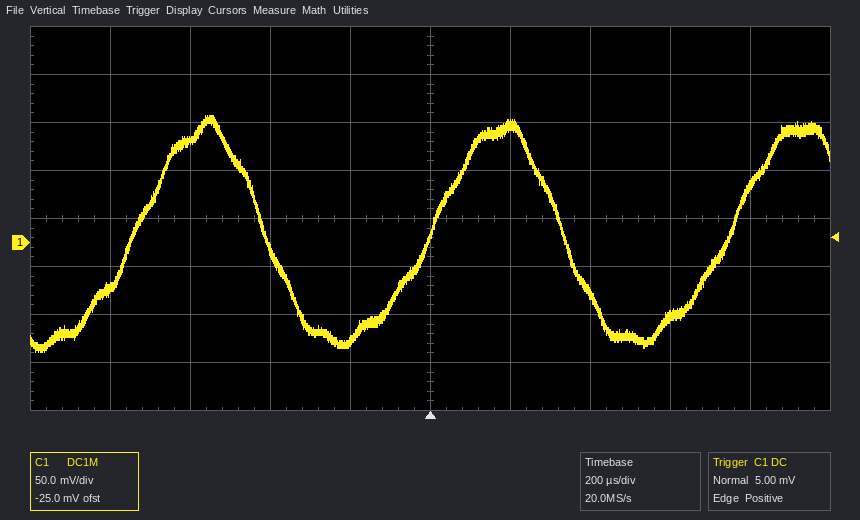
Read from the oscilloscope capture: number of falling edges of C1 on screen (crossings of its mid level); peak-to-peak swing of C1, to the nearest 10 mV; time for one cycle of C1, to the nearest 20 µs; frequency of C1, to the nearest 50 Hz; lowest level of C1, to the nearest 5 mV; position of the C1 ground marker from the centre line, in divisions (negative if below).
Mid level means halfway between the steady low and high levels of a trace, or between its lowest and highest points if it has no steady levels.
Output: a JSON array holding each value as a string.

["2", "250 mV", "740 µs", "1.35 kHz", "-115 mV", "-0.5 div"]
